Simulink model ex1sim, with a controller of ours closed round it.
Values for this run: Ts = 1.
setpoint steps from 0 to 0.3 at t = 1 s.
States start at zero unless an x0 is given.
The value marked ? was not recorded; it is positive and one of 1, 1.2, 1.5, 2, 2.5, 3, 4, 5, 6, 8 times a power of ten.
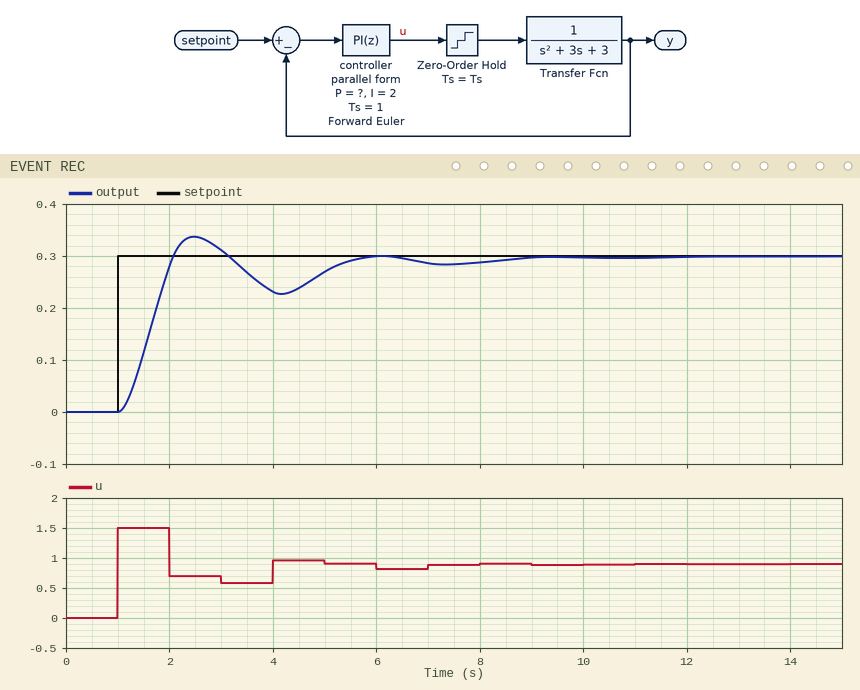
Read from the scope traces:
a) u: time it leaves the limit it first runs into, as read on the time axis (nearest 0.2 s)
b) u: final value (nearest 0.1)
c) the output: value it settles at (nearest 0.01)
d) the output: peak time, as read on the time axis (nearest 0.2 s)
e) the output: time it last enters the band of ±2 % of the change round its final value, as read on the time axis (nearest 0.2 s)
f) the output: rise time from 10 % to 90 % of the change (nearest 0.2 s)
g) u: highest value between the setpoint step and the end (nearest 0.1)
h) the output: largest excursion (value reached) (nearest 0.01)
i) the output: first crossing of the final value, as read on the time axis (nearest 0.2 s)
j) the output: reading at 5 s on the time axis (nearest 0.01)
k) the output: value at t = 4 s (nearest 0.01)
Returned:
2.0 s
0.9
0.30
2.4 s
8.6 s
0.8 s
1.5
0.34
2.0 s
0.27
0.23
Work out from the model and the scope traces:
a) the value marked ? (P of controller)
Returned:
5
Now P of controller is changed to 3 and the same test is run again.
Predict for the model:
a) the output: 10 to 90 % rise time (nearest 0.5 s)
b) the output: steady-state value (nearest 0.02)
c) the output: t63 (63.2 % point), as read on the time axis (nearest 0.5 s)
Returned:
1.5 s
0.30
2.0 s
